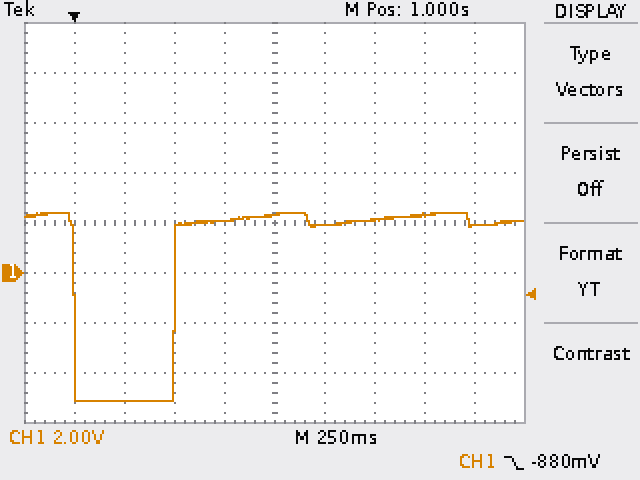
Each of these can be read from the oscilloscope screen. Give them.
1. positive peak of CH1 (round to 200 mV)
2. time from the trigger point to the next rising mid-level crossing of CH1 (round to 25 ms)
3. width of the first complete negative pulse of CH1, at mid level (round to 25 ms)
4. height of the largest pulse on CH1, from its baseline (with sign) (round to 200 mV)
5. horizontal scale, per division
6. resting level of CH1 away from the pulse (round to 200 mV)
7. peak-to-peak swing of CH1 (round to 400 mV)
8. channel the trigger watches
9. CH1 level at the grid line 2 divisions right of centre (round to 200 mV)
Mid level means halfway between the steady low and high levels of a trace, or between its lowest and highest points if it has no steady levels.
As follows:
2.4 V
500 ms
500 ms
-7.2 V
250 ms
2.0 V
7.6 V
CH1
2.2 V
